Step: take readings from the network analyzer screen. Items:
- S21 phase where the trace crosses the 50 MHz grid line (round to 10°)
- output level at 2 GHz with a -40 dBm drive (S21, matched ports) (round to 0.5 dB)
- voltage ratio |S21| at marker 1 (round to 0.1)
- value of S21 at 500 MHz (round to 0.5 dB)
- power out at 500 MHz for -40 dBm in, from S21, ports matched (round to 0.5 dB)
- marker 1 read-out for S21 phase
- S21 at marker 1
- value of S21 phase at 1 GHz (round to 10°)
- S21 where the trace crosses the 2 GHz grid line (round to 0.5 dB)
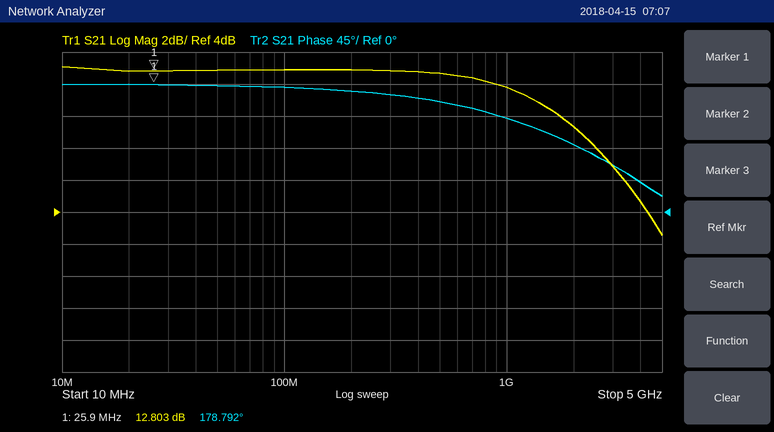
180°
-30.5 dBm
4.4
12.5 dB
-27.5 dBm
178.792°
12.803 dB
130°
9.5 dB
